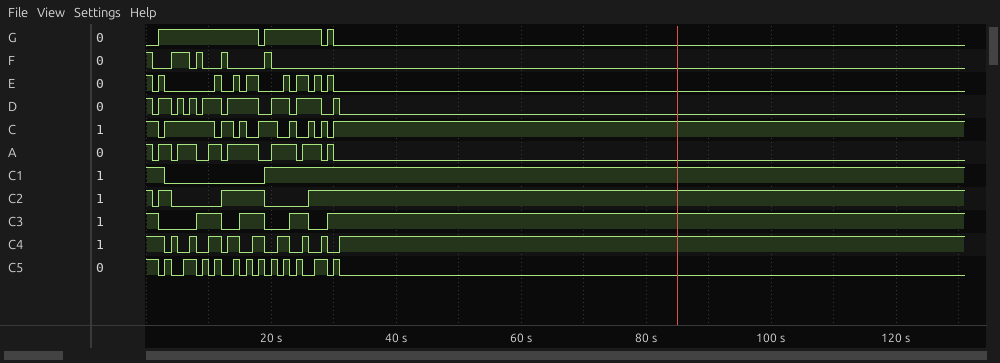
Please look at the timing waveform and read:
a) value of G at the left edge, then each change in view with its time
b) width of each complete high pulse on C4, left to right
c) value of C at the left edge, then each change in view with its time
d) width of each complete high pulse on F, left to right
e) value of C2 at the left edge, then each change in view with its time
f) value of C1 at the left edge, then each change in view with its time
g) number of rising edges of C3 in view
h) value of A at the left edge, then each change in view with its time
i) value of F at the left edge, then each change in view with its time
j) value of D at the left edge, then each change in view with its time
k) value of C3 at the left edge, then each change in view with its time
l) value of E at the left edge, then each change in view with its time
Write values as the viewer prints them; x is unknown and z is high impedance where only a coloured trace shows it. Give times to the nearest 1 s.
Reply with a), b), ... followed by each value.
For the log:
a) 0, 1 at 2 s, 0 at 18 s, 1 at 19 s, 0 at 28 s, 1 at 29 s, 0 at 30 s
b) 1 s, 1 s, 2 s, 2 s, 2 s, 2 s, 1 s, 1 s
c) 1, 0 at 2 s, 1 at 3 s, 0 at 11 s, 1 at 12 s, 0 at 14 s, 1 at 15 s, 0 at 16 s, 1 at 18 s, 0 at 21 s, 1 at 23 s, 0 at 24 s, 1 at 26 s, 0 at 27 s, 1 at 28 s, 0 at 29 s, 1 at 30 s
d) 3 s, 1 s, 1 s, 1 s
e) 1, 0 at 1 s, 1 at 2 s, 0 at 4 s, 1 at 12 s, 0 at 19 s, 1 at 26 s
f) 1, 0 at 3 s, 1 at 19 s
g) 4
h) 1, 0 at 1 s, 1 at 2 s, 0 at 4 s, 1 at 5 s, 0 at 8 s, 1 at 10 s, 0 at 12 s, 1 at 13 s, 0 at 18 s, 1 at 20 s, 0 at 24 s, 1 at 25 s, 0 at 28 s, 1 at 29 s, 0 at 30 s
i) 1, 0 at 1 s, 1 at 4 s, 0 at 7 s, 1 at 8 s, 0 at 9 s, 1 at 12 s, 0 at 13 s, 1 at 19 s, 0 at 20 s
j) 1, 0 at 1 s, 1 at 2 s, 0 at 4 s, 1 at 5 s, 0 at 6 s, 1 at 7 s, 0 at 8 s, 1 at 9 s, 0 at 12 s, 1 at 13 s, 0 at 18 s, 1 at 20 s, 0 at 23 s, 1 at 24 s, 0 at 28 s, 1 at 30 s, 0 at 31 s
k) 1, 0 at 2 s, 1 at 8 s, 0 at 12 s, 1 at 15 s, 0 at 19 s, 1 at 23 s, 0 at 26 s, 1 at 29 s
l) 1, 0 at 1 s, 1 at 2 s, 0 at 3 s, 1 at 11 s, 0 at 12 s, 1 at 14 s, 0 at 15 s, 1 at 16 s, 0 at 18 s, 1 at 22 s, 0 at 23 s, 1 at 24 s, 0 at 26 s, 1 at 27 s, 0 at 28 s, 1 at 29 s, 0 at 30 s
